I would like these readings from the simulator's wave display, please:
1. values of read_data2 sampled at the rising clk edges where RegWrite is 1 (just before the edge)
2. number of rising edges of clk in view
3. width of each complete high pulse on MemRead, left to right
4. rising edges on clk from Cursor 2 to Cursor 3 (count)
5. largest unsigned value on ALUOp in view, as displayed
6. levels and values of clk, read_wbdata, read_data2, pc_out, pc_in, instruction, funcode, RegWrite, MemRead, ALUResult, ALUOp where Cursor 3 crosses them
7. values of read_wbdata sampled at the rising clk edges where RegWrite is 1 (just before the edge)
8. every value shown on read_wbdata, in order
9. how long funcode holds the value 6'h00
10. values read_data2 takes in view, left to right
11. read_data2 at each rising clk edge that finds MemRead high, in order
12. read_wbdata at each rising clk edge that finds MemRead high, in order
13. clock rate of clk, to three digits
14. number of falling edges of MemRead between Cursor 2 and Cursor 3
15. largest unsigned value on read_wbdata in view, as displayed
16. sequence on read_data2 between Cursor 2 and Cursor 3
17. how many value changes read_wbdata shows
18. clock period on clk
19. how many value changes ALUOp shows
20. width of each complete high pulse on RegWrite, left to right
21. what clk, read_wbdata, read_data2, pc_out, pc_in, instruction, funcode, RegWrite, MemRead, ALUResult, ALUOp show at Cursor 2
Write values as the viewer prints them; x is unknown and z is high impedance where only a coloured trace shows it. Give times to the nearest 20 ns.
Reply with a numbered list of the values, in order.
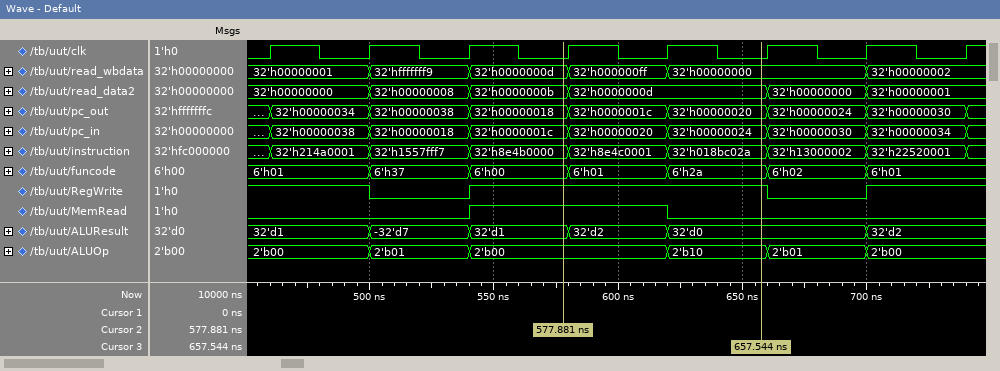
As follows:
1. 32'h00000000, 32'h00000000, 32'h0000000b, 32'h0000000d, 32'h0000000d, 32'h00000001
2. 8
3. 80 ns
4. 2
5. 2'b10
6. clk=0, read_wbdata=32'h00000000, read_data2=32'h0000000d, pc_out=32'h00000020, pc_in=32'h00000024, instruction=32'h018bc02a, funcode=6'h2a, RegWrite=1, MemRead=0, ALUResult=32'd0, ALUOp=2'b10
7. 32'h00000001, 32'h00000001, 32'h0000000d, 32'h000000ff, 32'h00000000, 32'h00000002
8. 32'h00000001, 32'hfffffff9, 32'h0000000d, 32'h000000ff, 32'h00000000, 32'h00000002
9. 40 ns
10. 32'h00000000, 32'h00000008, 32'h0000000b, 32'h0000000d, 32'h00000000, 32'h00000001
11. 32'h0000000b, 32'h0000000d
12. 32'h0000000d, 32'h000000ff
13. 25.0 MHz
14. 1
15. 32'hfffffff9
16. 32'h0000000b, 32'h0000000d
17. 5
18. 40 ns
19. 5
20. 120 ns
21. clk=0, read_wbdata=32'h0000000d, read_data2=32'h0000000b, pc_out=32'h00000018, pc_in=32'h0000001c, instruction=32'h8e4b0000, funcode=6'h00, RegWrite=1, MemRead=1, ALUResult=32'd1, ALUOp=2'b00
